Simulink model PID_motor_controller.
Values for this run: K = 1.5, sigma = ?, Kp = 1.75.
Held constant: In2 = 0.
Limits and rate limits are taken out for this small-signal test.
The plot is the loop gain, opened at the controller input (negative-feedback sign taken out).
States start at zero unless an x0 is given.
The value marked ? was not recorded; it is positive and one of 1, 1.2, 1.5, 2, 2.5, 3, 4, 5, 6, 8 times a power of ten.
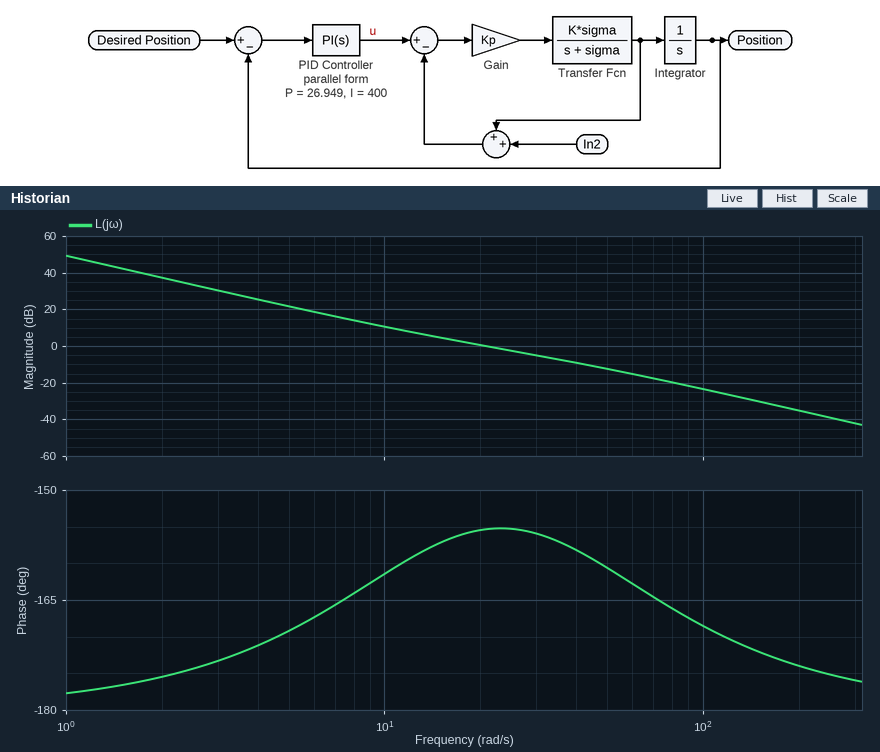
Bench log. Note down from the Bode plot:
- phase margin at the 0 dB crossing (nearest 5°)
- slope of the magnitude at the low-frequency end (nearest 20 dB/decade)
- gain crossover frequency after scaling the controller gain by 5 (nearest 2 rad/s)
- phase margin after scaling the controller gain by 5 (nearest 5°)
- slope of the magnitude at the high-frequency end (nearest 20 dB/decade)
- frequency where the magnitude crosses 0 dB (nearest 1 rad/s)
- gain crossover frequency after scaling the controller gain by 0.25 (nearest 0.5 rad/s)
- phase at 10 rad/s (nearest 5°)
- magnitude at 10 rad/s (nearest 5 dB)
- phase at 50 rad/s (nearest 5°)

25°
-40 dB/decade
56 rad/s
20°
-40 dB/decade
21 rad/s
9.0 rad/s
-160°
10 dB
-160°
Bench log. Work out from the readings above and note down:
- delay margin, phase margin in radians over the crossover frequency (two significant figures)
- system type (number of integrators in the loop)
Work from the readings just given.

0.021 s
2
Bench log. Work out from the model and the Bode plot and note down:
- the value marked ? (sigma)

10
